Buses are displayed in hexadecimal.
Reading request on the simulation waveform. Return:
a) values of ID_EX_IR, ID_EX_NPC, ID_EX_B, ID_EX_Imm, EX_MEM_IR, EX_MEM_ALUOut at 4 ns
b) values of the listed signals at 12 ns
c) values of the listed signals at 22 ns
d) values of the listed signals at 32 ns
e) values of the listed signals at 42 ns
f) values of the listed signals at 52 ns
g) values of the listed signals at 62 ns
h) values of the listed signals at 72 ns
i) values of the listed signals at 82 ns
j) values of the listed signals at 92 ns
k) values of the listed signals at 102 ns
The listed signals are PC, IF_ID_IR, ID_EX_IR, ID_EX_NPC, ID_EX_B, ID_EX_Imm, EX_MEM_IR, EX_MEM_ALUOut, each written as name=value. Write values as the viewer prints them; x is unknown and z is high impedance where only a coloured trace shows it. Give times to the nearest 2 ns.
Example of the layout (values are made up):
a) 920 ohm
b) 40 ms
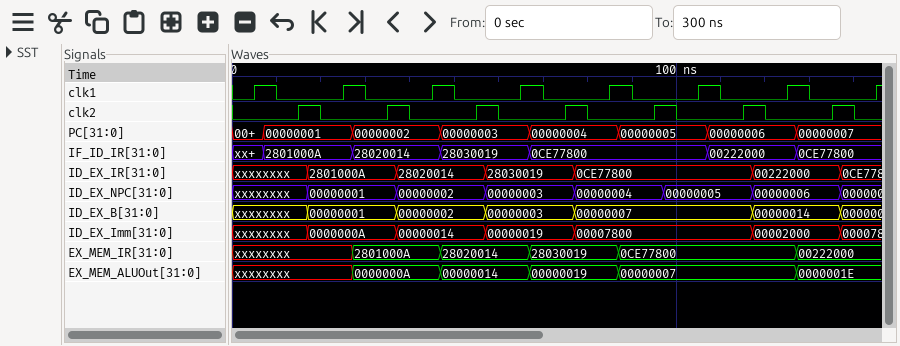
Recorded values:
a) ID_EX_IR=xxxxxxxx, ID_EX_NPC=xxxxxxxx, ID_EX_B=xxxxxxxx, ID_EX_Imm=xxxxxxxx, EX_MEM_IR=xxxxxxxx, EX_MEM_ALUOut=xxxxxxxx
b) PC=00000001, IF_ID_IR=2801000A, ID_EX_IR=xxxxxxxx, ID_EX_NPC=xxxxxxxx, ID_EX_B=xxxxxxxx, ID_EX_Imm=xxxxxxxx, EX_MEM_IR=xxxxxxxx, EX_MEM_ALUOut=xxxxxxxx
c) PC=00000001, IF_ID_IR=2801000A, ID_EX_IR=2801000A, ID_EX_NPC=00000001, ID_EX_B=00000001, ID_EX_Imm=0000000A, EX_MEM_IR=xxxxxxxx, EX_MEM_ALUOut=xxxxxxxx
d) PC=00000002, IF_ID_IR=28020014, ID_EX_IR=2801000A, ID_EX_NPC=00000001, ID_EX_B=00000001, ID_EX_Imm=0000000A, EX_MEM_IR=2801000A, EX_MEM_ALUOut=0000000A
e) PC=00000002, IF_ID_IR=28020014, ID_EX_IR=28020014, ID_EX_NPC=00000002, ID_EX_B=00000002, ID_EX_Imm=00000014, EX_MEM_IR=2801000A, EX_MEM_ALUOut=0000000A
f) PC=00000003, IF_ID_IR=28030019, ID_EX_IR=28020014, ID_EX_NPC=00000002, ID_EX_B=00000002, ID_EX_Imm=00000014, EX_MEM_IR=28020014, EX_MEM_ALUOut=00000014
g) PC=00000003, IF_ID_IR=28030019, ID_EX_IR=28030019, ID_EX_NPC=00000003, ID_EX_B=00000003, ID_EX_Imm=00000019, EX_MEM_IR=28020014, EX_MEM_ALUOut=00000014
h) PC=00000004, IF_ID_IR=0CE77800, ID_EX_IR=28030019, ID_EX_NPC=00000003, ID_EX_B=00000003, ID_EX_Imm=00000019, EX_MEM_IR=28030019, EX_MEM_ALUOut=00000019
i) PC=00000004, IF_ID_IR=0CE77800, ID_EX_IR=0CE77800, ID_EX_NPC=00000004, ID_EX_B=00000007, ID_EX_Imm=00007800, EX_MEM_IR=28030019, EX_MEM_ALUOut=00000019
j) PC=00000005, IF_ID_IR=0CE77800, ID_EX_IR=0CE77800, ID_EX_NPC=00000004, ID_EX_B=00000007, ID_EX_Imm=00007800, EX_MEM_IR=0CE77800, EX_MEM_ALUOut=00000007
k) PC=00000005, IF_ID_IR=0CE77800, ID_EX_IR=0CE77800, ID_EX_NPC=00000005, ID_EX_B=00000007, ID_EX_Imm=00007800, EX_MEM_IR=0CE77800, EX_MEM_ALUOut=00000007
